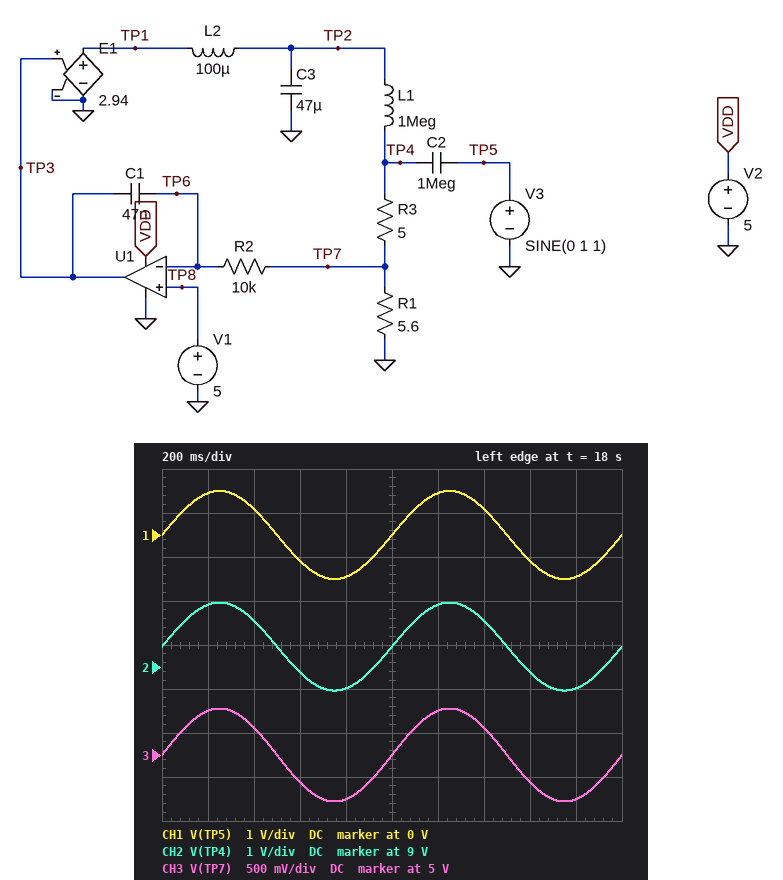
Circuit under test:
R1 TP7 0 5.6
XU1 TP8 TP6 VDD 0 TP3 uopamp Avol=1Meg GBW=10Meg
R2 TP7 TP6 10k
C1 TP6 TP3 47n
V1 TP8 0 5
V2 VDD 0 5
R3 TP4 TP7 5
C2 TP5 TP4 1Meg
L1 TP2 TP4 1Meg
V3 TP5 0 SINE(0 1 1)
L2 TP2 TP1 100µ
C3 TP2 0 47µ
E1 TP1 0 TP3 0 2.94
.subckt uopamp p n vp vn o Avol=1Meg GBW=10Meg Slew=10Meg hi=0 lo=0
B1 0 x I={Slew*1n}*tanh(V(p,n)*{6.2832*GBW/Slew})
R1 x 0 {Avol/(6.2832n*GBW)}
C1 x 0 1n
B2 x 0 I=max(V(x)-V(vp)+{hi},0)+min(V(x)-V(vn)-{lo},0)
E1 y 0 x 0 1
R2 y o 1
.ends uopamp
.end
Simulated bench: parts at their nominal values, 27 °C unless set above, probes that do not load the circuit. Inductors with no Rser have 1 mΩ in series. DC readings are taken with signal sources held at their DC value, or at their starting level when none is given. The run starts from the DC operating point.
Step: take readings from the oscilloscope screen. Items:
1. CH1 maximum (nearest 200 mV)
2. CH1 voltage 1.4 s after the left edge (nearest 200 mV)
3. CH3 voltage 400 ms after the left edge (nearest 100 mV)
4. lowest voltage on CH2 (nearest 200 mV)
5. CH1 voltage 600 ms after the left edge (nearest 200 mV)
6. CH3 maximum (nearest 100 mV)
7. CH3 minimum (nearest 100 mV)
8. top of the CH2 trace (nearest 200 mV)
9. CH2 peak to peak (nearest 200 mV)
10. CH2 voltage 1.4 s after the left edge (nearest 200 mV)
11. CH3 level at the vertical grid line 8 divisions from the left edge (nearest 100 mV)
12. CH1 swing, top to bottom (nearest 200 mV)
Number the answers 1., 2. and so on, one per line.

1. 1.0 V
2. 600 mV
3. 5.3 V
4. 8.4 V
5. -600 mV
6. 5.5 V
7. 4.5 V
8. 10.4 V
9. 2.0 V
10. 10.0 V
11. 4.7 V
12. 2.0 V
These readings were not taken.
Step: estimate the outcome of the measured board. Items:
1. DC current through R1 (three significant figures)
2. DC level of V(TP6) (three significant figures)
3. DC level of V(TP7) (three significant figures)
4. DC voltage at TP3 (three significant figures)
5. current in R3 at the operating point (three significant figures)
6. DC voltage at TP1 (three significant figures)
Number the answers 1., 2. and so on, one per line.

1. 893 mA
2. 5.00 V
3. 5.00 V
4. 3.22 V
5. 893 mA
6. 9.47 V
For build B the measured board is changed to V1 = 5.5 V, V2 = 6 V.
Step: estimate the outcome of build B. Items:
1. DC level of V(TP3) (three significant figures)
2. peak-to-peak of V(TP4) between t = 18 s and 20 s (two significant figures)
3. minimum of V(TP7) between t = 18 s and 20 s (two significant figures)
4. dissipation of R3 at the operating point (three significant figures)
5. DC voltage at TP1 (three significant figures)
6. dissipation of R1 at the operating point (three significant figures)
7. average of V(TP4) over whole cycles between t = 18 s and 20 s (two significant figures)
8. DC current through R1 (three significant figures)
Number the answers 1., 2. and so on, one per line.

1. 3.54 V
2. 2.0 V
3. 5.0 V
4. 4.82 W
5. 10.4 V
6. 5.40 W
7. 10 V
8. 982 mA
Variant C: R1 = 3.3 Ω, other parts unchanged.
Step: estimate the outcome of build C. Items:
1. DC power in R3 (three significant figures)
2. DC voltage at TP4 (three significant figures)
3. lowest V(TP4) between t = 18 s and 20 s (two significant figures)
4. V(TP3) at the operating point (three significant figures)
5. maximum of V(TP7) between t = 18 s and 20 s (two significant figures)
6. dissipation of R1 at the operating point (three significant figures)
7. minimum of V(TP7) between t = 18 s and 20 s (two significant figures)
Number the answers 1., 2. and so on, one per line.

1. 11.5 W
2. 12.6 V
3. 12 V
4. 4.28 V
5. 5.4 V
6. 7.58 W
7. 4.6 V
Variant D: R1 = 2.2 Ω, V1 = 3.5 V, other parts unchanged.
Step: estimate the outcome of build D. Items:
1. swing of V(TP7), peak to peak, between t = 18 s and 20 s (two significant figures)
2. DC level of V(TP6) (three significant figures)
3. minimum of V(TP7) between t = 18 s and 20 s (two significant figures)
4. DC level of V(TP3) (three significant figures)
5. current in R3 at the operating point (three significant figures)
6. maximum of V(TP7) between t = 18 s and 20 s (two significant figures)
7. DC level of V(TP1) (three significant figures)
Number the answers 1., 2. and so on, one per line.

1. 610 mV
2. 3.50 V
3. 3.2 V
4. 3.90 V
5. 1.59 A
6. 3.8 V
7. 11.5 V
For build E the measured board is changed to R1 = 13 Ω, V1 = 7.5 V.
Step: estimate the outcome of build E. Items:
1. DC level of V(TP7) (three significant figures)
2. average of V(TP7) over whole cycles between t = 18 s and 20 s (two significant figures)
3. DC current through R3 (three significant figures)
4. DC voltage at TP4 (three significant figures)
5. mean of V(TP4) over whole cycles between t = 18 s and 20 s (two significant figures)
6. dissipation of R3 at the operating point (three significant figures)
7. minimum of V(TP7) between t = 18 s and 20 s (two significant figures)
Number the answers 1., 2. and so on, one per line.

1. 7.50 V
2. 7.5 V
3. 577 mA
4. 10.4 V
5. 10 V
6. 1.66 W
7. 6.8 V
